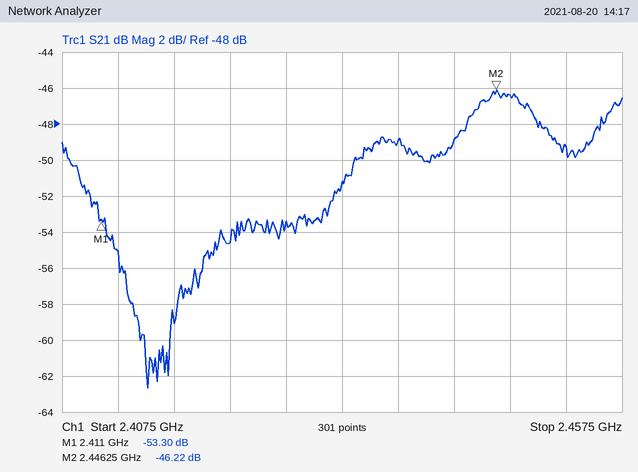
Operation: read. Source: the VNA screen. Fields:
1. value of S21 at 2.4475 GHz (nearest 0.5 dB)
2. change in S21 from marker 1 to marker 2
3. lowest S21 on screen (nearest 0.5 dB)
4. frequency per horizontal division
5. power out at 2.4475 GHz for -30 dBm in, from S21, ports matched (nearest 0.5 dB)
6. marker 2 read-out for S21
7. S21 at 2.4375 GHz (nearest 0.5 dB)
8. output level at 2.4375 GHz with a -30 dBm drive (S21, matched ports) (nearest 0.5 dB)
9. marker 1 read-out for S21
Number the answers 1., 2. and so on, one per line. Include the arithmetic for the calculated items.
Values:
1. -46.5 dB
2. -46.22 − (-53.3) = 7.08 dB
3. -62.5 dB
4. 5 MHz
5. -30 dBm + (-46.5 dB) = -76.5 dBm
6. -46.22 dB
7. -49.0 dB
8. -30 dBm + (-49.0 dB) = -79.0 dBm
9. -53.30 dB
